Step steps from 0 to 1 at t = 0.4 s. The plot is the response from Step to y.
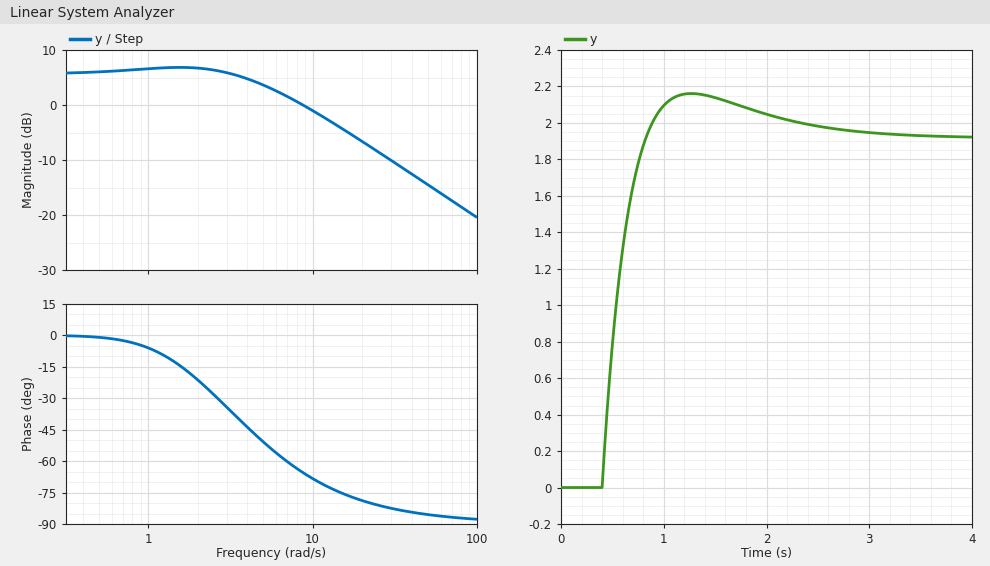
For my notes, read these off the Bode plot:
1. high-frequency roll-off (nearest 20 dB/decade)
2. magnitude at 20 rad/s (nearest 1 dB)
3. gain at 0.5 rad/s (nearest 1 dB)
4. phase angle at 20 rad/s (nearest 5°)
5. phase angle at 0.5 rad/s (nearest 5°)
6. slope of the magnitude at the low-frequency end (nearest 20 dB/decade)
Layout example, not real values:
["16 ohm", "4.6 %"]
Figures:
["-20 dB/decade", "-7 dB", "6 dB", "-80°", "0°", "0 dB/decade"]
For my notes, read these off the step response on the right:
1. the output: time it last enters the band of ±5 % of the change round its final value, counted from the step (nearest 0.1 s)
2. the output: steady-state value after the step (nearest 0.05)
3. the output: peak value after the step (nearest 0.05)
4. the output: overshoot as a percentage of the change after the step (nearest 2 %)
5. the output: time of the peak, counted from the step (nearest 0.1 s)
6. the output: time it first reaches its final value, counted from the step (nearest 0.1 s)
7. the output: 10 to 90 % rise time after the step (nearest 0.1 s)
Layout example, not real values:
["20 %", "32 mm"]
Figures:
["1.8 s", "1.90", "2.15", "12 %", "0.9 s", "0.4 s", "0.3 s"]
